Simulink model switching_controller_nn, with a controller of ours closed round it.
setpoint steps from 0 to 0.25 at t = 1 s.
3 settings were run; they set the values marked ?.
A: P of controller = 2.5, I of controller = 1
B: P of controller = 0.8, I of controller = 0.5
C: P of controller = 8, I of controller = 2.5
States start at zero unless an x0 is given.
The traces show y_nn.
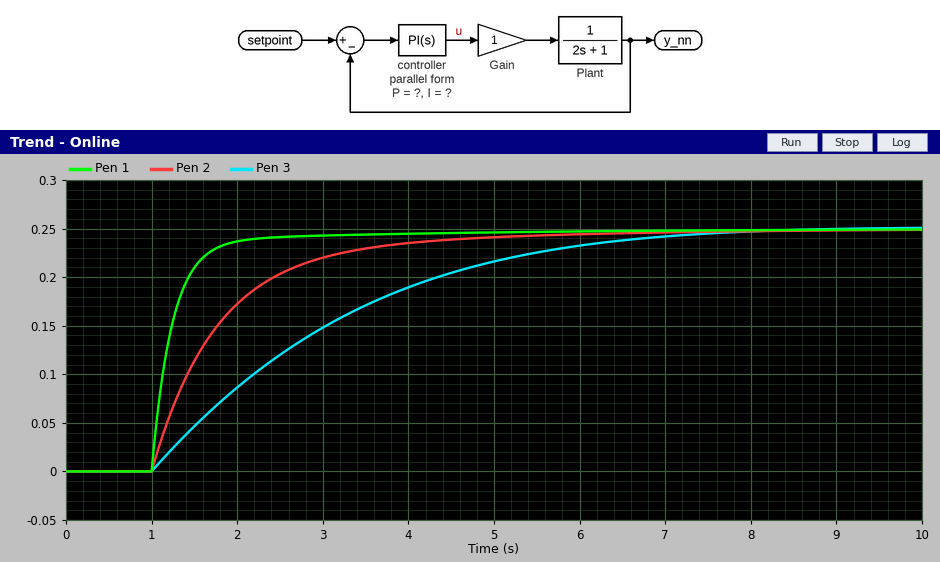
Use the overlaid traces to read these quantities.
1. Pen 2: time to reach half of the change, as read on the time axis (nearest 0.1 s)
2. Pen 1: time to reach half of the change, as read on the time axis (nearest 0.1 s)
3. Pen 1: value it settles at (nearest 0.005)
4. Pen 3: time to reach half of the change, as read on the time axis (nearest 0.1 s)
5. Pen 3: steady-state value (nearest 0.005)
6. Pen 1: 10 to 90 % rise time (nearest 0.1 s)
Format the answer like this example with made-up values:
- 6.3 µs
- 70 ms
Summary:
- 1.6 s
- 1.2 s
- 0.250
- 2.6 s
- 0.250
- 0.6 s
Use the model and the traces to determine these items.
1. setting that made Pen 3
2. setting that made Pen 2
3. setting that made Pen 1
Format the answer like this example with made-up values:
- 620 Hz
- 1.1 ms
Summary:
- B
- A
- C
